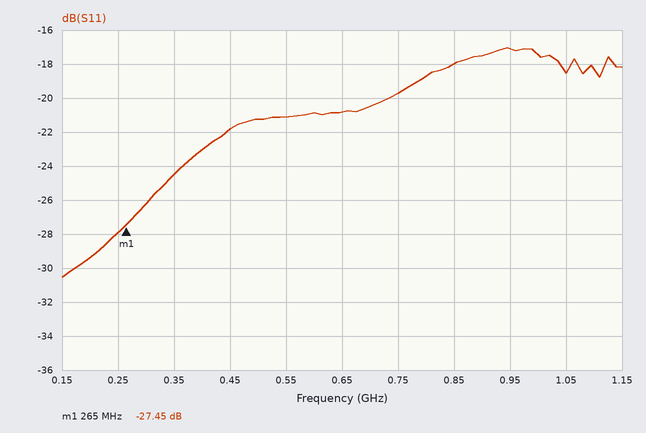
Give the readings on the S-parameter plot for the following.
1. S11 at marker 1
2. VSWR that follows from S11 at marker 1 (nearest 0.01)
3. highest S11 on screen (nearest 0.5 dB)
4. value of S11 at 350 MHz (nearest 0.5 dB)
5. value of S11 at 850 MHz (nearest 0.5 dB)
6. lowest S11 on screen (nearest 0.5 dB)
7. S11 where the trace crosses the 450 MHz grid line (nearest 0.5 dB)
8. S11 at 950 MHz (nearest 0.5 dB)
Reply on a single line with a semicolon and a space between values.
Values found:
-27.45 dB; 1.09; -17.0 dB; -24.5 dB; -18.0 dB; -30.5 dB; -22.0 dB; -17.0 dB
